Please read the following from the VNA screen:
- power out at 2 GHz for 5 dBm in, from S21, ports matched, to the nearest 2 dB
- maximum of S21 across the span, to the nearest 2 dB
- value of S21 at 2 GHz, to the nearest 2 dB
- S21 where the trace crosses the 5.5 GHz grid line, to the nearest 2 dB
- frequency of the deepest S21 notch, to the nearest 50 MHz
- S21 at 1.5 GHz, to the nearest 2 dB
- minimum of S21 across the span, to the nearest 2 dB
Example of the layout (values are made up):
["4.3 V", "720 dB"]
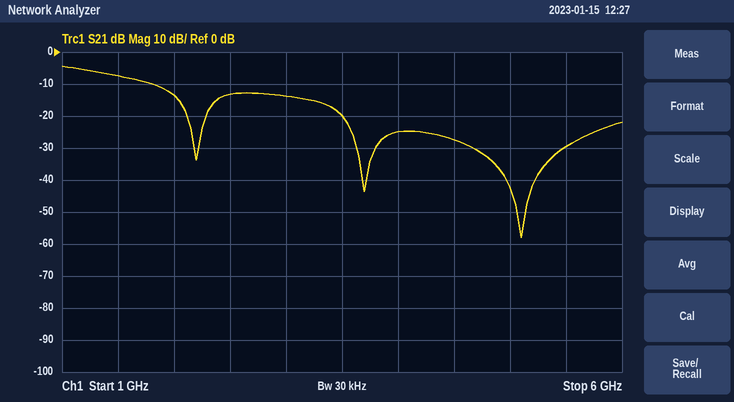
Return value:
["-8 dBm", "-4 dB", "-14 dB", "-30 dB", "5.10 GHz", "-8 dB", "-58 dB"]
